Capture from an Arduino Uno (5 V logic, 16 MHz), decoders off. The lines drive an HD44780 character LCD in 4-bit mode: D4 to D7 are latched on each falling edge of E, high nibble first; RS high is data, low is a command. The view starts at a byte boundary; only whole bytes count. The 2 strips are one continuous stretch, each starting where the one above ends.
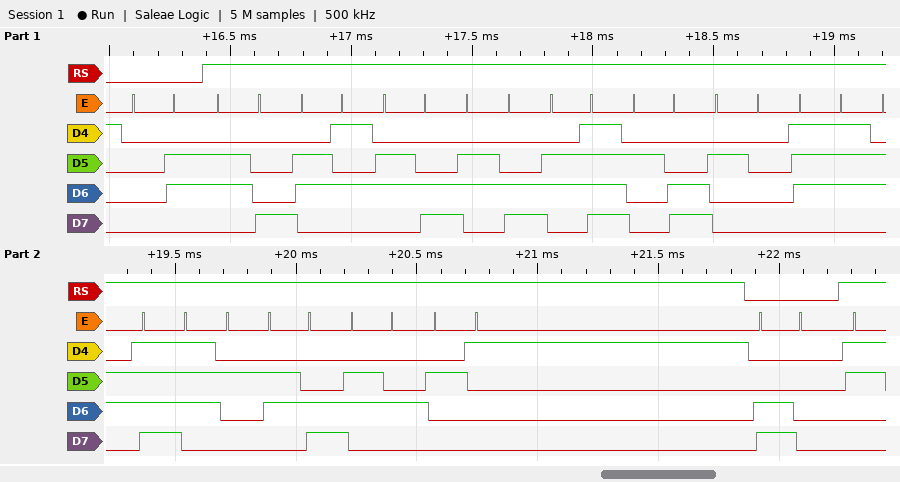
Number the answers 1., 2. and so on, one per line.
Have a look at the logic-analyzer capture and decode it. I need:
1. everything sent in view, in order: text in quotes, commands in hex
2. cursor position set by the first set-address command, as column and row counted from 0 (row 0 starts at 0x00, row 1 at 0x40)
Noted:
1. 0x06 "hello, world!" 0xC0
2. column 0, row 1
